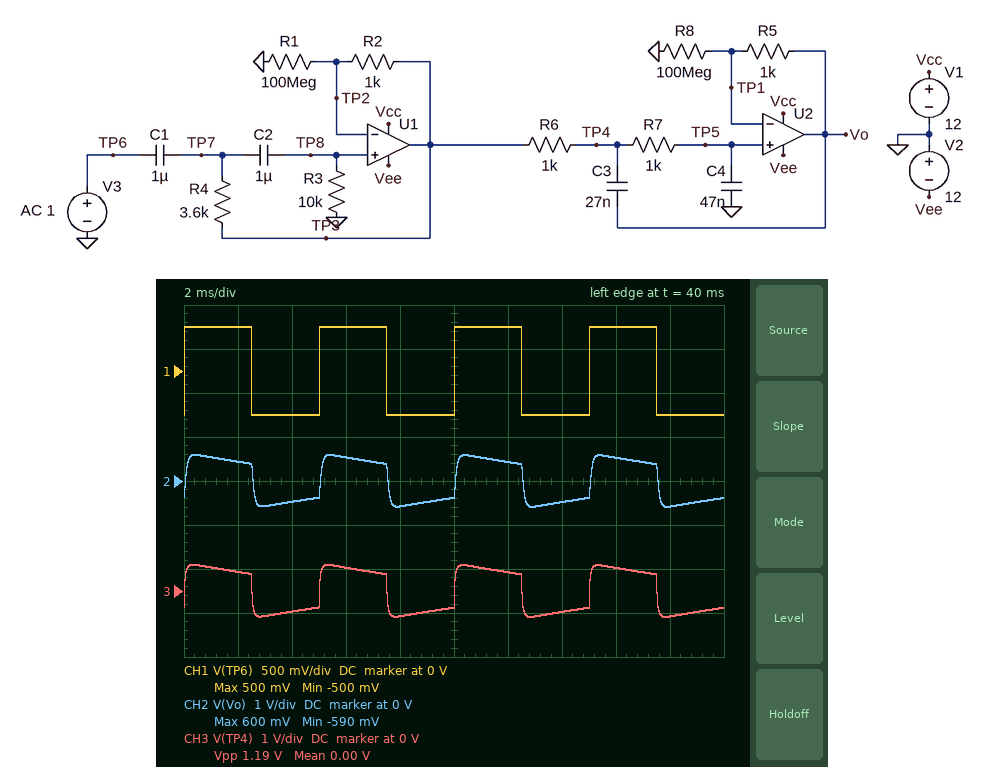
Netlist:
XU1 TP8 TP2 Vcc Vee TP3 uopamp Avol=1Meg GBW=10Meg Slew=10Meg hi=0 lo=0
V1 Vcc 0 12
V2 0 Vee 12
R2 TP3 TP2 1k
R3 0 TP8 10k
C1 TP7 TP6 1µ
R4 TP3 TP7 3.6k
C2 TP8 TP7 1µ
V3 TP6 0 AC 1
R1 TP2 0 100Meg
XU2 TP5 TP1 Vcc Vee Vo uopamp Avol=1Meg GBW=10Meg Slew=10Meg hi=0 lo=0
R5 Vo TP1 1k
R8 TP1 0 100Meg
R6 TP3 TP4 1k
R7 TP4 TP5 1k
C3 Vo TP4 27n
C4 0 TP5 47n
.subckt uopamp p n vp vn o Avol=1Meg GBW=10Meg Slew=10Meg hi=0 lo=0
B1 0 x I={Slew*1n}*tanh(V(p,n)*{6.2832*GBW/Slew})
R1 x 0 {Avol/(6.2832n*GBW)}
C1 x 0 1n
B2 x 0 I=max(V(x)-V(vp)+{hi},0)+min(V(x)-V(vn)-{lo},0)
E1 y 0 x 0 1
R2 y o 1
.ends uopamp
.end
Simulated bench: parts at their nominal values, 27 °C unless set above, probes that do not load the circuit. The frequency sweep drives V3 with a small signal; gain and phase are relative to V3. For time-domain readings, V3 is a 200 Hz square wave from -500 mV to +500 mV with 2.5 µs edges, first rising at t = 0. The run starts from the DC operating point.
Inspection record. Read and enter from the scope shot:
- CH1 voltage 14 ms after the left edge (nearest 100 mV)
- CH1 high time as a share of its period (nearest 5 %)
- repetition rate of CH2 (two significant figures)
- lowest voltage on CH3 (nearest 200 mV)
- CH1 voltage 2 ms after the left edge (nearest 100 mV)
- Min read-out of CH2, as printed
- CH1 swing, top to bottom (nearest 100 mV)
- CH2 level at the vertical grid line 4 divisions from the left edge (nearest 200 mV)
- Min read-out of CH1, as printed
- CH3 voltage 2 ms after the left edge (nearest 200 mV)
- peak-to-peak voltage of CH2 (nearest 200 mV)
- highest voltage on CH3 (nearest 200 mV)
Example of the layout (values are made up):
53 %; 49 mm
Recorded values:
-500 mV; 50 %; 200 Hz; -600 mV; 500 mV; -590 mV; 1.0 V; -600 mV; -500 mV; 400 mV; 1.2 V; 600 mV
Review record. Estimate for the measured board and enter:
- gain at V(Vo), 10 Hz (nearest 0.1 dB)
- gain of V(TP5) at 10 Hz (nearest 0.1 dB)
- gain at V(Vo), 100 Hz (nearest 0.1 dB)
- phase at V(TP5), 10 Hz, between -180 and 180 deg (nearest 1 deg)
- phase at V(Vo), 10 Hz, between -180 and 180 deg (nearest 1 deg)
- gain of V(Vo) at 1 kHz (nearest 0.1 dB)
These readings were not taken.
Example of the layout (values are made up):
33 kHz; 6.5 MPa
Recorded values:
-16.7 dB; -16.7 dB; 0.1 dB; 152 deg; 152 deg; -1.0 dB
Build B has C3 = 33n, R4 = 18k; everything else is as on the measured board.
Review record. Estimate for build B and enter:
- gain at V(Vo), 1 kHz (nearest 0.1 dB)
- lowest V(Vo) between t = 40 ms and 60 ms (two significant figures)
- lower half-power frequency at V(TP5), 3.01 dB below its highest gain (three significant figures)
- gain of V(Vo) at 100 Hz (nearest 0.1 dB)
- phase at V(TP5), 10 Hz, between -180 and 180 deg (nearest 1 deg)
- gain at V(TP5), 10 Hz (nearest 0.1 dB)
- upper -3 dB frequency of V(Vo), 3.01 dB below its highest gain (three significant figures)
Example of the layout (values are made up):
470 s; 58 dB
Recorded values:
-0.9 dB; -610 mV; 26.9 Hz; -0.3 dB; 97 deg; -10.1 dB; 2.08 kHz
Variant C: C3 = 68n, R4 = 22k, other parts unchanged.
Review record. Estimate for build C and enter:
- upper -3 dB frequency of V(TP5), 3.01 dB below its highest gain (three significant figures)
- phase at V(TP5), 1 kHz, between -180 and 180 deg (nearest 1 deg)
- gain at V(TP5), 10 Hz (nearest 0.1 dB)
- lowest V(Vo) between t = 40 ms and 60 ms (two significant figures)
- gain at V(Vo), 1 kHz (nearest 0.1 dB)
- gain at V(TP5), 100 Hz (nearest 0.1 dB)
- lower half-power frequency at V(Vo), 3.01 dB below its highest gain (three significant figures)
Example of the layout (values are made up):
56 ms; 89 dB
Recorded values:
2.36 kHz; -32 deg; -10.1 dB; -640 mV; -0.5 dB; -0.3 dB; 27.8 Hz
